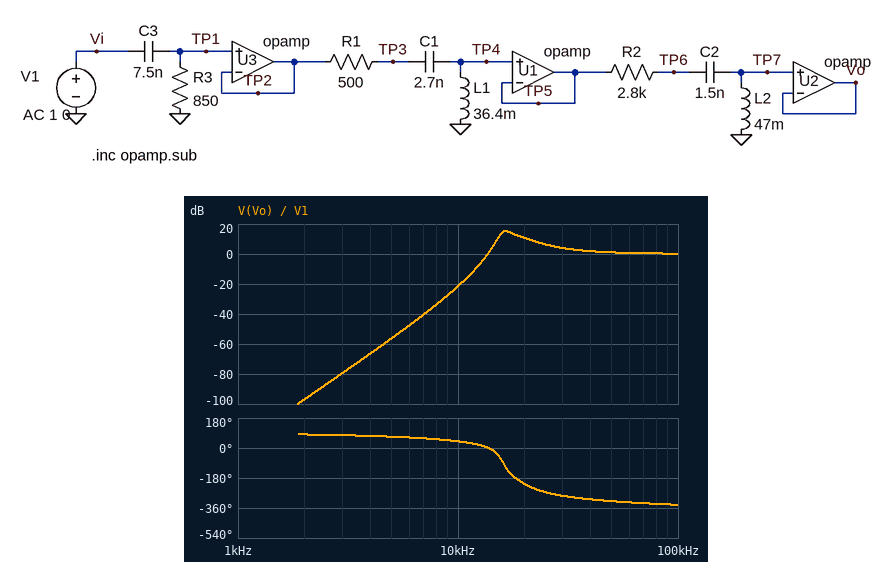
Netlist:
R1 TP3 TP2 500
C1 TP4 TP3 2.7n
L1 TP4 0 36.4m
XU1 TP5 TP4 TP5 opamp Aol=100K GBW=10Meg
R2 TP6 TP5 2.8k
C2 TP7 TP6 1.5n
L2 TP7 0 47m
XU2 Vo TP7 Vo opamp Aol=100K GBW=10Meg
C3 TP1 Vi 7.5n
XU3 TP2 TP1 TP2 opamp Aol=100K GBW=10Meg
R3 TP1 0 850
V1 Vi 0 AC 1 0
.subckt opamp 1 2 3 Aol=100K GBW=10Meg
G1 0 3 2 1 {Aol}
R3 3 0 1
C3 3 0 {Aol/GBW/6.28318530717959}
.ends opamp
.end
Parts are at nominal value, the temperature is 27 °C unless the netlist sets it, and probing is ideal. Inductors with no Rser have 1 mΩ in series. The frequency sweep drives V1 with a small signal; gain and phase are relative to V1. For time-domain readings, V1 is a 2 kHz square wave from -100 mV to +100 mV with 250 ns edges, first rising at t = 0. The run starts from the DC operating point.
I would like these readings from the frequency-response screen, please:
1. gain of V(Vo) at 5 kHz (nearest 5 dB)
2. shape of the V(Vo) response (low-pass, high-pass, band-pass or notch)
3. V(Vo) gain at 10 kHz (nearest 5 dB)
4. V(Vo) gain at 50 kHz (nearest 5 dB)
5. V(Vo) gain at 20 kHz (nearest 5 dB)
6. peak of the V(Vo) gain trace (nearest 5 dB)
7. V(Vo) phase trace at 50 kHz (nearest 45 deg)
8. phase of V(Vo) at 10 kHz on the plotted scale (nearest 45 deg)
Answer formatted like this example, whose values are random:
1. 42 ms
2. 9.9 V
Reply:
1. -55 dB
2. high-pass
3. -20 dB
4. 0 dB
5. 10 dB
6. 15 dB
7. -315 deg
8. 45 deg
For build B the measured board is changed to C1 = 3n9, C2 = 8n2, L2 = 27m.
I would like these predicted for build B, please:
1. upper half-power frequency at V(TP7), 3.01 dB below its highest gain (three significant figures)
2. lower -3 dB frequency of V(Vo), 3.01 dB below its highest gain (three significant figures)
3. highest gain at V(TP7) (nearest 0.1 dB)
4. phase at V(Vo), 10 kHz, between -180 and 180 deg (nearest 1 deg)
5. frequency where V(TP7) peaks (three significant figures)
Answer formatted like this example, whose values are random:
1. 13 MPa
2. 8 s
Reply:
1. 15.2 kHz
2. 12.6 kHz
3. 7.2 dB
4. -33 deg
5. 13.6 kHz
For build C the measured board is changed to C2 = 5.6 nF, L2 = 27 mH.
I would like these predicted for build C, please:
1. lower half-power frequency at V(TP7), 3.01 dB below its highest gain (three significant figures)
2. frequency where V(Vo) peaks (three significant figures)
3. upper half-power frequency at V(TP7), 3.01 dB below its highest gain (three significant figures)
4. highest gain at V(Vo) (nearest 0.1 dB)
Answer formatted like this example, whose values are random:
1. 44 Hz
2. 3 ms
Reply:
1. 15.3 kHz
2. 16.2 kHz
3. 17.6 kHz
4. 11.4 dB
